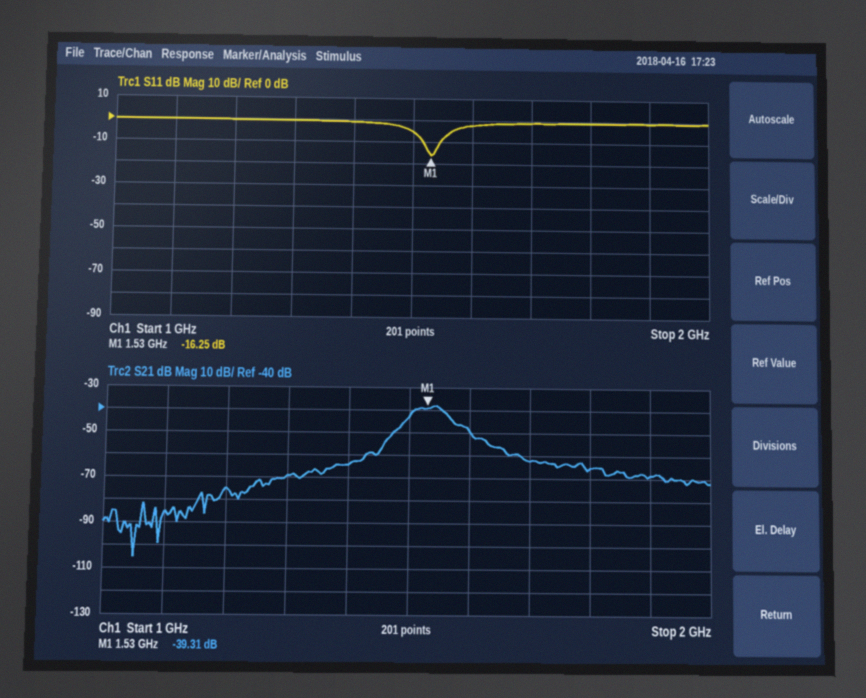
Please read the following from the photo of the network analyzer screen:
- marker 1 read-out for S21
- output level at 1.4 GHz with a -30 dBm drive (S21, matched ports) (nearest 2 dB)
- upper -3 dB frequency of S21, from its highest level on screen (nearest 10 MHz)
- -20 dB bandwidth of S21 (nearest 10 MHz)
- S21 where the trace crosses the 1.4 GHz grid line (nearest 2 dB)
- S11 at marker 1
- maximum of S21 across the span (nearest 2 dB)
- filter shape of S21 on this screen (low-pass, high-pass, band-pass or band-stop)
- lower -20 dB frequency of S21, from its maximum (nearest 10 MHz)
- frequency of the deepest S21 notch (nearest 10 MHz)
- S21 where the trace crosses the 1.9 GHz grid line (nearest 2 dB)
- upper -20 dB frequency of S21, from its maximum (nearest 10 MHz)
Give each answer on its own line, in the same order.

-39.31 dB
-94 dBm
1.56 GHz
210 MHz
-64 dB
-16.25 dB
-38 dB
band-pass
1.45 GHz
1.05 GHz
-68 dB
1.66 GHz
